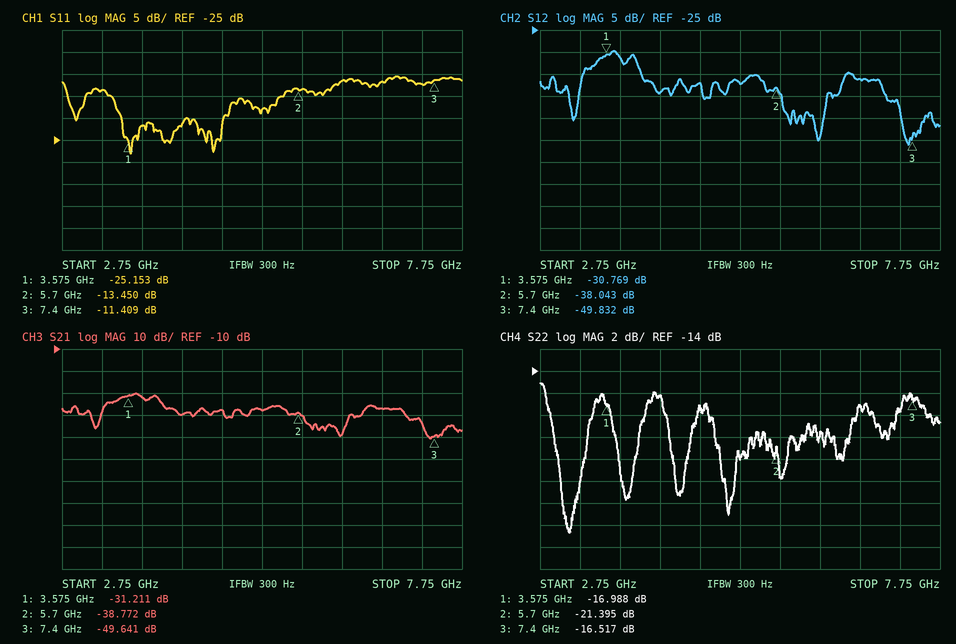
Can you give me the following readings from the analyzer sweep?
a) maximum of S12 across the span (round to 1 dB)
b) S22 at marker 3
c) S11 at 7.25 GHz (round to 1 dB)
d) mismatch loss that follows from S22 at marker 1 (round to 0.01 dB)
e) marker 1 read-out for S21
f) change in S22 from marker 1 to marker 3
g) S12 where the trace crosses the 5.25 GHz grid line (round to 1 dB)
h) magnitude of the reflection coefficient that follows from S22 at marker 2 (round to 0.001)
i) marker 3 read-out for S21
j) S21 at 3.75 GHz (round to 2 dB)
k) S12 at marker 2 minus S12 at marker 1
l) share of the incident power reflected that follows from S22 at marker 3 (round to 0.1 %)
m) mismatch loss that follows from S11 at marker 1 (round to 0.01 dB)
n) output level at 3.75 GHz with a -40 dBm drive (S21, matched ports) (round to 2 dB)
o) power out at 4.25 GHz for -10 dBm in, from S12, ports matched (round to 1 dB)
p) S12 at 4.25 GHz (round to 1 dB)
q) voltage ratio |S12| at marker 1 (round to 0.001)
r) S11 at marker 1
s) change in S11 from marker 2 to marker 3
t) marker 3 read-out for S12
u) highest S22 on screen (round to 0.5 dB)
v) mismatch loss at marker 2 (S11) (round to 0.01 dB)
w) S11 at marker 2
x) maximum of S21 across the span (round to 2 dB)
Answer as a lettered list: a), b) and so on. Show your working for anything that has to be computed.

a) -30 dB
b) -16.517 dB
c) -12 dB
d) −10 log10(1 − 10^(-16.988/10)) ≈ 0.09 dB
e) -31.211 dB
f) -16.517 − (-16.988) = 0.471 dB
g) -37 dB
h) 10^(-21.395/20) ≈ 0.085
i) -49.641 dB
j) -32 dB
k) -38.043 − (-30.769) = -7.274 dB
l) 10^(-16.517/10) ≈ 2.2 %
m) −10 log10(1 − 10^(-25.153/10)) ≈ 0.01 dB
n) -40 dBm + (-32 dB) = -72 dBm
o) -10 dBm + (-39 dB) = -49 dBm
p) -39 dB
q) 10^(-30.769/20) ≈ 0.029
r) -25.153 dB
s) -11.409 − (-13.45) = 2.041 dB
t) -49.832 dB
u) -15.0 dB
v) −10 log10(1 − 10^(-13.45/10)) ≈ 0.20 dB
w) -13.450 dB
x) -30 dB
